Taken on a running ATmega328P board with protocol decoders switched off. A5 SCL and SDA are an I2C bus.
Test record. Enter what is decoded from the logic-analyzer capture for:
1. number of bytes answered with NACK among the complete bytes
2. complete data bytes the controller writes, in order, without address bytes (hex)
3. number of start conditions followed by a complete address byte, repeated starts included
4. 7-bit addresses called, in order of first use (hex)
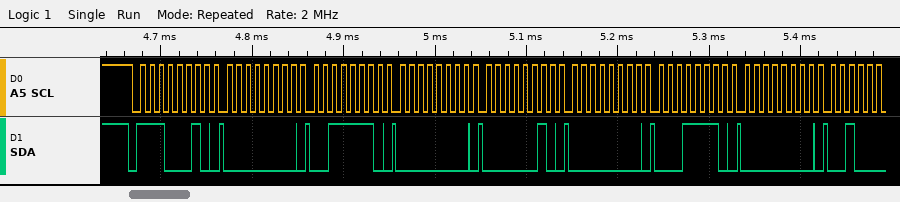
0
00 3E 00 02 00 1E 00
1
0x71
